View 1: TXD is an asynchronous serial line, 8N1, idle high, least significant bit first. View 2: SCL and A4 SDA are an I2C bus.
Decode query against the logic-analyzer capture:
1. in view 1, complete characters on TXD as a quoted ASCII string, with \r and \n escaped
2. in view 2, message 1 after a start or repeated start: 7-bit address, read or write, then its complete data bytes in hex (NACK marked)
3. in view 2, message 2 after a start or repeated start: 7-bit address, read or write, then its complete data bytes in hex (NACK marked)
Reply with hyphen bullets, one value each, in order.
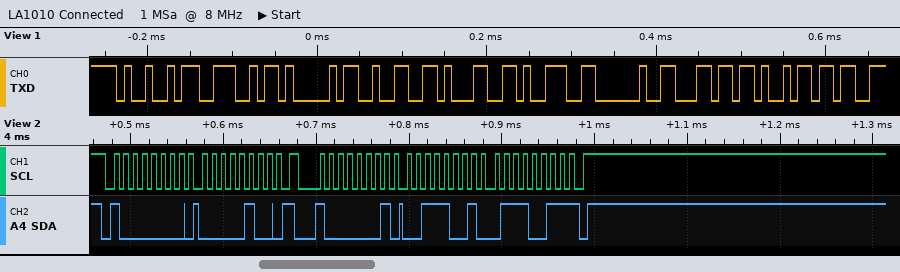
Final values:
- "INA219 li"
- 0x40 write: 04
- 0x40 read: 39 73 NACK
